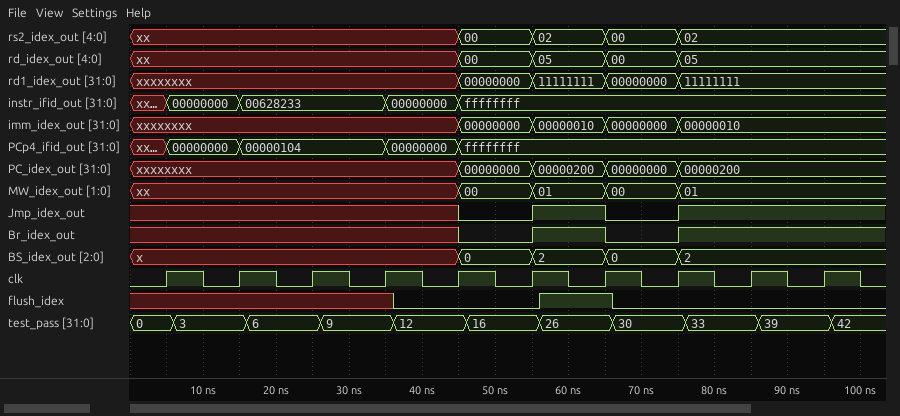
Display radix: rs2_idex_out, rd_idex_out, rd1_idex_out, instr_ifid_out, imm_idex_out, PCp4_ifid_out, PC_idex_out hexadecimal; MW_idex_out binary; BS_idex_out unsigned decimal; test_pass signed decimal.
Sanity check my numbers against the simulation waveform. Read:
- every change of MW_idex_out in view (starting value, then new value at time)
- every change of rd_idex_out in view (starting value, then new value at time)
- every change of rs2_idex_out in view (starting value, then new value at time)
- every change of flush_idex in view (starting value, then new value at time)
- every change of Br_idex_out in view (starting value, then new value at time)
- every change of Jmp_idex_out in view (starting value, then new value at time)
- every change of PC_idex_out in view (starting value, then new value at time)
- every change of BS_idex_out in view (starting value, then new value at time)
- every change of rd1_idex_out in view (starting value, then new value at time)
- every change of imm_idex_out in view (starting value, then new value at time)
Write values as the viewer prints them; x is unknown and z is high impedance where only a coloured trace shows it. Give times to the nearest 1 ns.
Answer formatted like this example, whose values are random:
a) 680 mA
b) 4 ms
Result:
a) xx, 00 at 45 ns, 01 at 55 ns, 00 at 65 ns, 01 at 75 ns
b) xx, 00 at 45 ns, 05 at 55 ns, 00 at 65 ns, 05 at 75 ns
c) xx, 00 at 45 ns, 02 at 55 ns, 00 at 65 ns, 02 at 75 ns
d) x, 0 at 36 ns, 1 at 56 ns, 0 at 66 ns
e) x, 0 at 45 ns, 1 at 55 ns, 0 at 65 ns, 1 at 75 ns
f) x, 0 at 45 ns, 1 at 55 ns, 0 at 65 ns, 1 at 75 ns
g) xxxxxxxx, 00000000 at 45 ns, 00000200 at 55 ns, 00000000 at 65 ns, 00000200 at 75 ns
h) x, 0 at 45 ns, 2 at 55 ns, 0 at 65 ns, 2 at 75 ns
i) xxxxxxxx, 00000000 at 45 ns, 11111111 at 55 ns, 00000000 at 65 ns, 11111111 at 75 ns
j) xxxxxxxx, 00000000 at 45 ns, 00000010 at 55 ns, 00000000 at 65 ns, 00000010 at 75 ns
